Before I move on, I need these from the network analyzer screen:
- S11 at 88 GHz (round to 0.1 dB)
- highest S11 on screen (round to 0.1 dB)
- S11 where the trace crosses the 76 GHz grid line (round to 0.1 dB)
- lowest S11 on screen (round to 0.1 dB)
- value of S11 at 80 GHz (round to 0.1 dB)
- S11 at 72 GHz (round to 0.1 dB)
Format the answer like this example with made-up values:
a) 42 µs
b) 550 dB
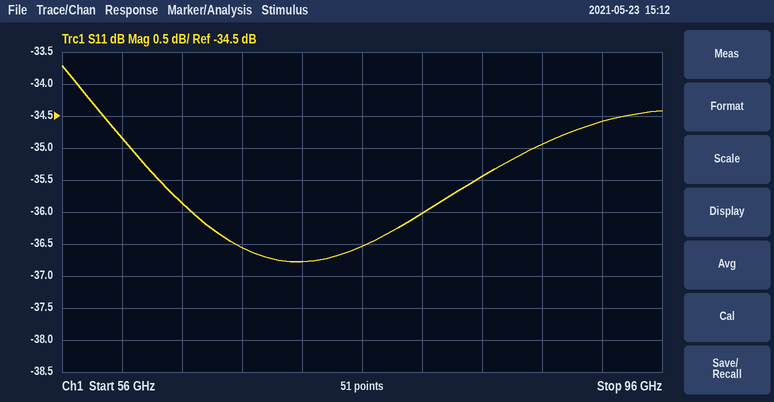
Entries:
a) -34.9 dB
b) -33.7 dB
c) -36.5 dB
d) -36.8 dB
e) -36.0 dB
f) -36.8 dB
